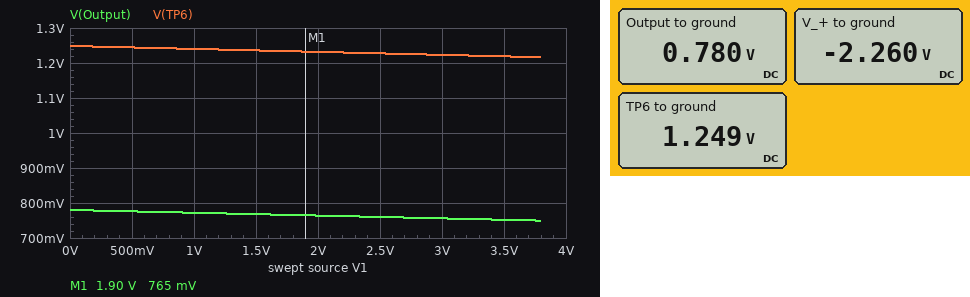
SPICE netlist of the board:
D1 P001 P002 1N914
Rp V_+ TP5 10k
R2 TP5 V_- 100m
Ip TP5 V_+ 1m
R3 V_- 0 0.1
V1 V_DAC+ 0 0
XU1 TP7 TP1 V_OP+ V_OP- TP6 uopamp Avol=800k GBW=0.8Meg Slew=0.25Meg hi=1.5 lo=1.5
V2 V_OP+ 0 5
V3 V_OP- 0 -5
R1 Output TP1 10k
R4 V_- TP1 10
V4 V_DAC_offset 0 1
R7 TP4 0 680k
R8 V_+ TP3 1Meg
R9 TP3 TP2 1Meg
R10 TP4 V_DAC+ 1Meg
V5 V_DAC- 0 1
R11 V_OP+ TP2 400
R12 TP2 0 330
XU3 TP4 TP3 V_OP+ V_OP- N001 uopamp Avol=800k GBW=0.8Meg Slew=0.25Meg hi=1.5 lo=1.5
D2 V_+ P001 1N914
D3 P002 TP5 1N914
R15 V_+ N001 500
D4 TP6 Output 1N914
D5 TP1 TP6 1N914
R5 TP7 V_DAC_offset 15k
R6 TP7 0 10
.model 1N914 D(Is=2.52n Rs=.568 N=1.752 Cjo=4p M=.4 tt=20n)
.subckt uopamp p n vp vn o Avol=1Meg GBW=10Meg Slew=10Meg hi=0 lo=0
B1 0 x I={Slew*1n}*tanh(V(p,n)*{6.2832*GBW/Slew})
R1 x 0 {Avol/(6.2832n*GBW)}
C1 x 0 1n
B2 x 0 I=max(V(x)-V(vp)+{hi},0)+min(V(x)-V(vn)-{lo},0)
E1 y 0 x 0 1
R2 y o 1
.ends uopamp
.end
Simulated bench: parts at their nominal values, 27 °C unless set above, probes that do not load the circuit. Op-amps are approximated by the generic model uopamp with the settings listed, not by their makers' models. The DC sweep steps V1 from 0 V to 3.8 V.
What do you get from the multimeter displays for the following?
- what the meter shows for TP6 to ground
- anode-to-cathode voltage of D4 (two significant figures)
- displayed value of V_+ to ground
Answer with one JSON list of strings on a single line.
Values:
["1.249 V", "470 mV", "-2.260 V"]
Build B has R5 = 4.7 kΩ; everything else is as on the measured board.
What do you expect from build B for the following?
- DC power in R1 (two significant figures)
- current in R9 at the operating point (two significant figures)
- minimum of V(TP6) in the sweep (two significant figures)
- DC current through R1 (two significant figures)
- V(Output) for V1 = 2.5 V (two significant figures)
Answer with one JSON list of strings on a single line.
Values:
["490 µW", "2.3 µA", "2.7 V", "220 µA", "2.2 V"]
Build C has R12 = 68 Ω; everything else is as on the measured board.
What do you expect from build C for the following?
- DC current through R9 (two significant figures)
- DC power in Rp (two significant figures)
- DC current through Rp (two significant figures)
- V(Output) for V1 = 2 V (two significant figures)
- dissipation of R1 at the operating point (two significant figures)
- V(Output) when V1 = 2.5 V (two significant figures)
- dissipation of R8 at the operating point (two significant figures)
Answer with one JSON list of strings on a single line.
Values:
["730 nA", "53 µW", "73 µA", "750 mV", "58 µW", "740 mV", "530 nW"]
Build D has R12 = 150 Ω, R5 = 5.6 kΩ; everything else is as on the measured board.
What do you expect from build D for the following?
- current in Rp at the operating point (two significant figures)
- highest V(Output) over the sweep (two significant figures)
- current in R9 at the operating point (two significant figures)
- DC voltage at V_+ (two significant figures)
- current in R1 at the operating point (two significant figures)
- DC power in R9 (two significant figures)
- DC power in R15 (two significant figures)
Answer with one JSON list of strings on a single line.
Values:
["140 µA", "1.9 V", "1.4 µA", "-1.4 V", "190 µA", "1.9 µW", "650 µW"]
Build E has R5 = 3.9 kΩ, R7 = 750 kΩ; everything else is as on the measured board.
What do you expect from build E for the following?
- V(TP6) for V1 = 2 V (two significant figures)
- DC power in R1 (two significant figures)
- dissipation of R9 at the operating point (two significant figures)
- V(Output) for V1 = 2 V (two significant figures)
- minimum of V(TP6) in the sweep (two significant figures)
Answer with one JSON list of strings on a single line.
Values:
["3.2 V", "700 µW", "5.1 µW", "2.6 V", "3.1 V"]
